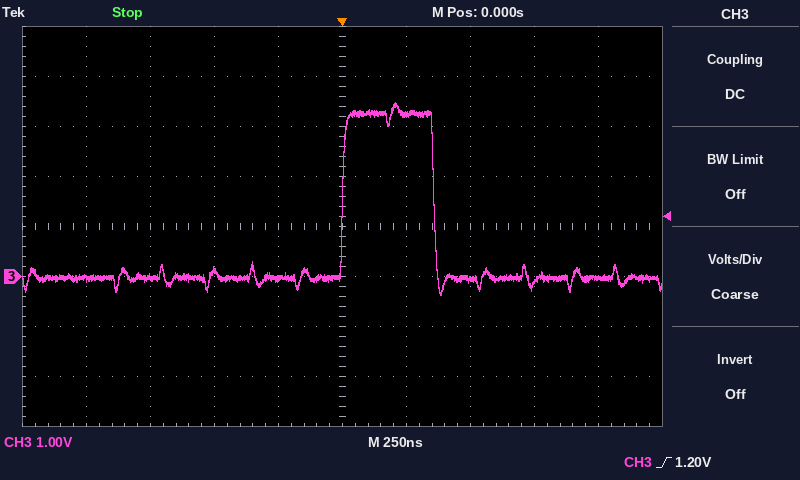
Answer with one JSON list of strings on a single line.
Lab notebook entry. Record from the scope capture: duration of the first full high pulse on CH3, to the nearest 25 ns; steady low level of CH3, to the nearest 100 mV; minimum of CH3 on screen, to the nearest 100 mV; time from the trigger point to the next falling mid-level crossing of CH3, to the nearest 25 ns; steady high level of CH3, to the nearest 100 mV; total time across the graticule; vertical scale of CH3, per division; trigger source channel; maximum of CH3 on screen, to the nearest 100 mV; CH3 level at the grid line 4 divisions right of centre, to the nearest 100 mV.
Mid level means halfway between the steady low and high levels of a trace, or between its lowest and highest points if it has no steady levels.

["350 ns", "0.0 V", "-400 mV", "350 ns", "3.3 V", "2.5 µs", "1 V", "CH3", "3.5 V", "0.0 V"]
